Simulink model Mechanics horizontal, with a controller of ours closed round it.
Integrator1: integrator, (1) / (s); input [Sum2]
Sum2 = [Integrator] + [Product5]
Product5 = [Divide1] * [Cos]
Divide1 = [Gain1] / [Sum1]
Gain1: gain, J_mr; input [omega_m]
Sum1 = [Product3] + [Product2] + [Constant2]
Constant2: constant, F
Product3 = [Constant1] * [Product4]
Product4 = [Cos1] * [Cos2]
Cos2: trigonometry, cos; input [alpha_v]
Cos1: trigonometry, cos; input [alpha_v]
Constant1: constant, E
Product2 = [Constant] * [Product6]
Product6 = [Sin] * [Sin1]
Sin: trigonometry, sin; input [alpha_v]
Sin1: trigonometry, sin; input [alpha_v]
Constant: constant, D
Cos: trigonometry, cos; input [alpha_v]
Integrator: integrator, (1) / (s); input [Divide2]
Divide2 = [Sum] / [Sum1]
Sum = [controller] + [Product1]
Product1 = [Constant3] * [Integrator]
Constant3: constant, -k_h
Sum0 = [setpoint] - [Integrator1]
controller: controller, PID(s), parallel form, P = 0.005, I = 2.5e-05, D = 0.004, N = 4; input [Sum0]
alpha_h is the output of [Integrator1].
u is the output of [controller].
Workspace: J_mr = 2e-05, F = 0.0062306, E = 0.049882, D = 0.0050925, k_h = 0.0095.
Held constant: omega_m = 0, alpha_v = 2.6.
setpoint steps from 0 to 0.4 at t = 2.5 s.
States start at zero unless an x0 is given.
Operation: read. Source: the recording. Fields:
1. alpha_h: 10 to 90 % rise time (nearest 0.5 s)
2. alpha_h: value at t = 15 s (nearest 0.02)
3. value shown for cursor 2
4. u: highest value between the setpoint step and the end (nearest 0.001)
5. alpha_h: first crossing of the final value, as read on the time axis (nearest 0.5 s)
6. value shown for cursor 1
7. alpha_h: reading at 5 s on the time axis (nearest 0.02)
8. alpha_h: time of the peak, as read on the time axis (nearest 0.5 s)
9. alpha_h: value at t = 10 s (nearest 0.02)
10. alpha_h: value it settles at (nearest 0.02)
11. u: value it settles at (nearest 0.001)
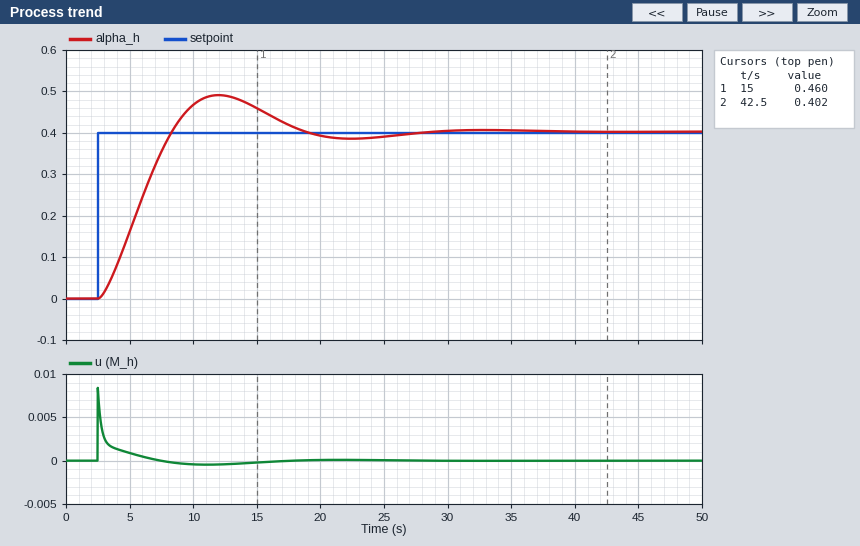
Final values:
4.0 s
0.46
0.402
0.008
8.5 s
0.460
0.16
12.0 s
0.46
0.40
0.000
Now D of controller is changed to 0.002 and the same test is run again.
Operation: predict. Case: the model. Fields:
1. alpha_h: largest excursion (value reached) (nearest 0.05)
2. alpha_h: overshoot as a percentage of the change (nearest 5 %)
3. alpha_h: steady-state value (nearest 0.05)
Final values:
0.50
30 %
0.40
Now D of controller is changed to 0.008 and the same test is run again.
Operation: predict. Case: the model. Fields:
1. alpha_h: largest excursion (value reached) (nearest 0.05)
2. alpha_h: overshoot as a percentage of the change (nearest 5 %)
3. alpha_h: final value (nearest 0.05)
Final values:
0.45
15 %
0.40
